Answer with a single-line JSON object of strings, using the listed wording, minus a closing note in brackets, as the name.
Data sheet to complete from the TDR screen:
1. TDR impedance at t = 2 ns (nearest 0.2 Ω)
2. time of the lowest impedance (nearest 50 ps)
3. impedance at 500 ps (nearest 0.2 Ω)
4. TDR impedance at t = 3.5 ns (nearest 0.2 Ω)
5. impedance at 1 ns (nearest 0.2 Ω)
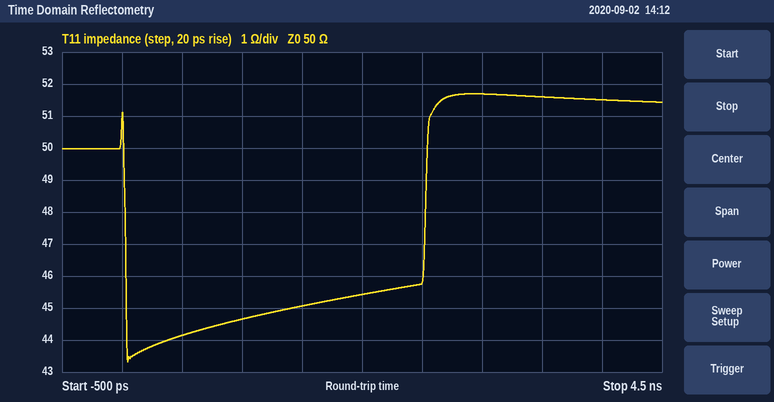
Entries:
{"TDR impedance at t = 2 ns": "45.4 Ω", "time of the lowest impedance": "50 ps", "impedance at 500 ps": "44.2 Ω", "TDR impedance at t = 3.5 ns": "51.6 Ω", "impedance at 1 ns": "44.6 Ω"}
